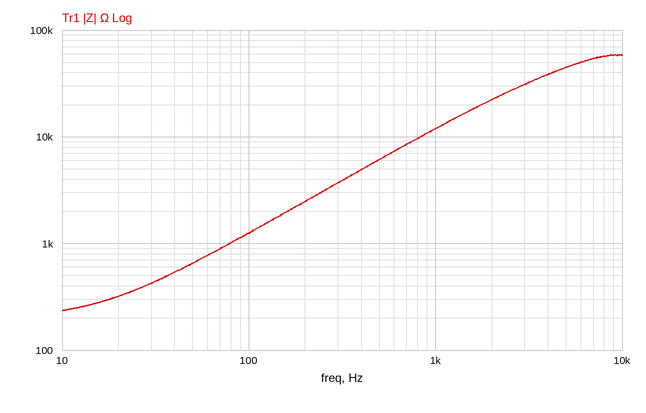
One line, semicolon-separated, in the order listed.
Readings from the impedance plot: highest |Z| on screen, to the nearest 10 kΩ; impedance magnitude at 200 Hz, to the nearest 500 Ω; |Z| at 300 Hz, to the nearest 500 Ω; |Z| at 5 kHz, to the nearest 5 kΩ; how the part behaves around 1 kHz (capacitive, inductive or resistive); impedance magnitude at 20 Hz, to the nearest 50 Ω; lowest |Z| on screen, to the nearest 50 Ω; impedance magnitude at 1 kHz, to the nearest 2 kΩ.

60 kΩ; 2.5 kΩ; 3.5 kΩ; 45 kΩ; inductive; 300 Ω; 250 Ω; 12 kΩ
